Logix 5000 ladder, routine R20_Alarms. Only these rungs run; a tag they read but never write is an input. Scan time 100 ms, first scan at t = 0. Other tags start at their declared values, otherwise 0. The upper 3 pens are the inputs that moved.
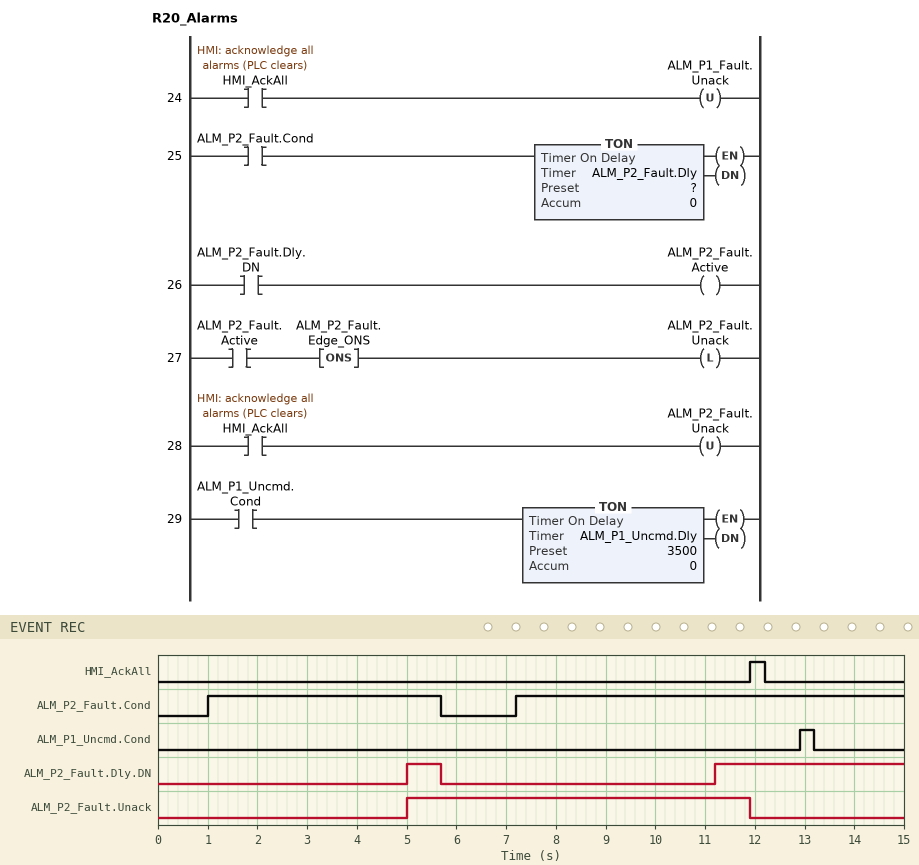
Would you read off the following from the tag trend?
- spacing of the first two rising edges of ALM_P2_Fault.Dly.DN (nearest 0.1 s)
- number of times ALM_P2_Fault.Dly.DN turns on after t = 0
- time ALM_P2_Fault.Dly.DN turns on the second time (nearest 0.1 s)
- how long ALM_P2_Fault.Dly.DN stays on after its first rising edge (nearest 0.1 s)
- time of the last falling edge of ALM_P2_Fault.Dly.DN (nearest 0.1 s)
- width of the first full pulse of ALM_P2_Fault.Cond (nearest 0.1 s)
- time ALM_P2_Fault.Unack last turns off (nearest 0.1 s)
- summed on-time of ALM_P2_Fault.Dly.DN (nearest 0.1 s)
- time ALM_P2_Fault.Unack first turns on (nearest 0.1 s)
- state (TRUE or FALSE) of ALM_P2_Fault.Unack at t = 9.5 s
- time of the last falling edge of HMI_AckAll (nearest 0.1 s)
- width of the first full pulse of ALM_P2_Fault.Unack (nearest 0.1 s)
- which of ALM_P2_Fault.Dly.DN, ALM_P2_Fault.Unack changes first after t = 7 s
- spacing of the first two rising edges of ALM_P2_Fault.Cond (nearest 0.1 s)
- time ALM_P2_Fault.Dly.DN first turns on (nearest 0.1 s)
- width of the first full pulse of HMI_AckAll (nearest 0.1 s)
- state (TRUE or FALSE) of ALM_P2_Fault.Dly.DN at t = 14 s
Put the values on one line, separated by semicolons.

6.2 s; 2; 11.2 s; 0.7 s; 5.7 s; 4.7 s; 11.9 s; 4.5 s; 5.0 s; TRUE; 12.2 s; 6.9 s; ALM_P2_Fault.Dly.DN; 6.2 s; 5.0 s; 0.3 s; TRUE
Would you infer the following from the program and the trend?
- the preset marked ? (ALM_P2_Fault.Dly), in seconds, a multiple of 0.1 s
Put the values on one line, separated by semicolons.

4.0 s
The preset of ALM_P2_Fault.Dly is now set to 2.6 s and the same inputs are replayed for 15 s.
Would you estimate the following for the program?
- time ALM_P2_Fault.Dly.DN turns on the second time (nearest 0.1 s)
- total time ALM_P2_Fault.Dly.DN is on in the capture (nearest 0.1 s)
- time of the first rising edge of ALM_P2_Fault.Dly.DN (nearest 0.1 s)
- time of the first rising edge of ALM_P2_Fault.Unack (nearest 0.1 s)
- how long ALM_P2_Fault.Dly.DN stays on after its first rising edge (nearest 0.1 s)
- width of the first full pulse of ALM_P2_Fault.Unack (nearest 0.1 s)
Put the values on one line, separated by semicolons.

9.8 s; 7.3 s; 3.6 s; 3.6 s; 2.1 s; 8.3 s
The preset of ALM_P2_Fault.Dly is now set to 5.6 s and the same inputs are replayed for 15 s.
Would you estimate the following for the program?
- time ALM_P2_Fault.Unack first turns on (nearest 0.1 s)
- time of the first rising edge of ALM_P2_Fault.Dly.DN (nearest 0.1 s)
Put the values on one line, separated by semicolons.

12.8 s; 12.8 s
